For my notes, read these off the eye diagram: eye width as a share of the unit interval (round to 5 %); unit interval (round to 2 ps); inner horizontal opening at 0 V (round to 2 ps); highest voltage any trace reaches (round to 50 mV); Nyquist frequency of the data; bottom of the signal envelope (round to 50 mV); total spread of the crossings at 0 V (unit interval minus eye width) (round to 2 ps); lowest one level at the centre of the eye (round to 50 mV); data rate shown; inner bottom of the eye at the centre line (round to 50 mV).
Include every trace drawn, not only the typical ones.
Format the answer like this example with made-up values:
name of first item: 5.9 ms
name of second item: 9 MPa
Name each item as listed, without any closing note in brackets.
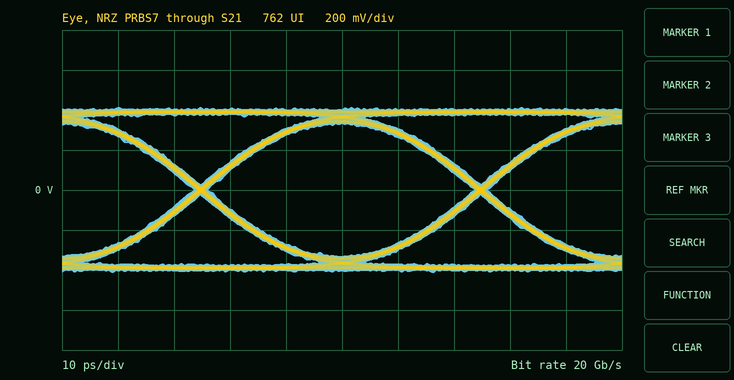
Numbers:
eye width as a share of the unit interval: 95 %
unit interval: 50 ps
inner horizontal opening at 0 V: 48 ps
highest voltage any trace reaches: 400 mV
Nyquist frequency of the data: 10 GHz
bottom of the signal envelope: -400 mV
total spread of the crossings at 0 V (unit interval minus eye width): 2 ps
lowest one level at the centre of the eye: 350 mV
data rate shown: 20 Gb/s
inner bottom of the eye at the centre line: -350 mV
